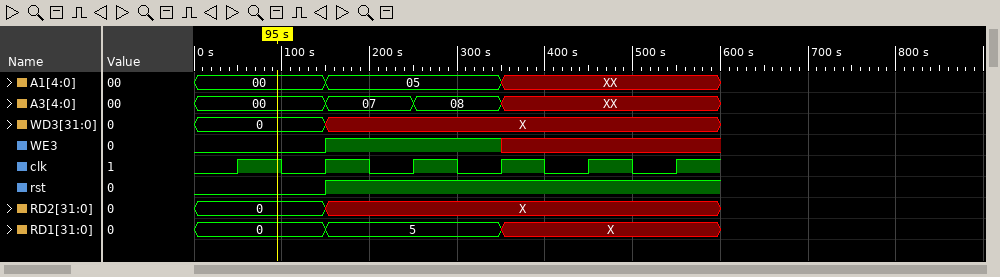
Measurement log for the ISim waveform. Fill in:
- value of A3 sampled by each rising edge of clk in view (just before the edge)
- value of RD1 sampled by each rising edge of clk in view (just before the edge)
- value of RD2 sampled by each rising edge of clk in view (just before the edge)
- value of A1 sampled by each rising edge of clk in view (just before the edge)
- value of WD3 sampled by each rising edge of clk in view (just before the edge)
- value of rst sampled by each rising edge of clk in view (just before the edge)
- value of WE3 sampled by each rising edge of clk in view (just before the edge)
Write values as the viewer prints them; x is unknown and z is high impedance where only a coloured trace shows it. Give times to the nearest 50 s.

00, 00, 07, 08, XX, XX
0, 0, 5, 5, X, X
0, 0, X, X, X, X
00, 00, 05, 05, XX, XX
0, 0, X, X, X, X
0 0 1 1 1 1
0 0 1 1 x x
